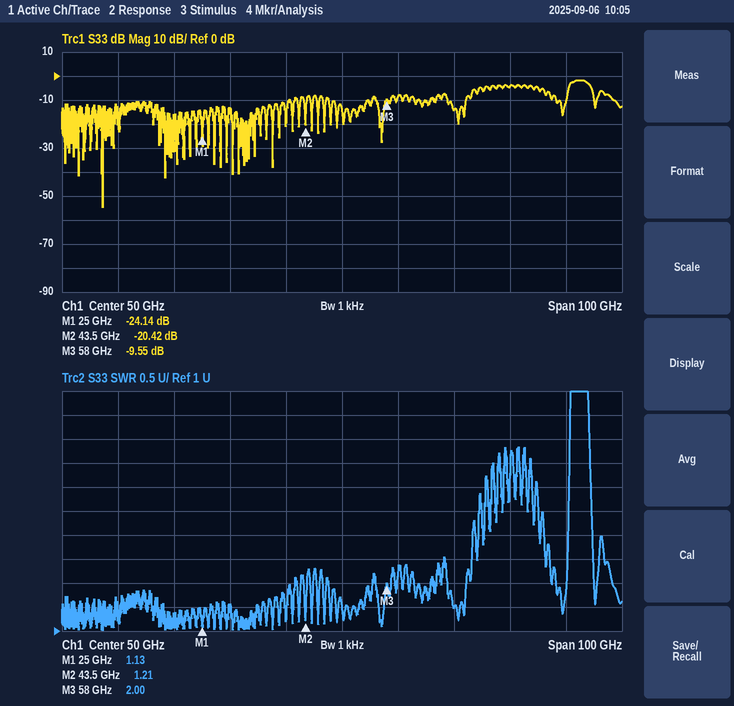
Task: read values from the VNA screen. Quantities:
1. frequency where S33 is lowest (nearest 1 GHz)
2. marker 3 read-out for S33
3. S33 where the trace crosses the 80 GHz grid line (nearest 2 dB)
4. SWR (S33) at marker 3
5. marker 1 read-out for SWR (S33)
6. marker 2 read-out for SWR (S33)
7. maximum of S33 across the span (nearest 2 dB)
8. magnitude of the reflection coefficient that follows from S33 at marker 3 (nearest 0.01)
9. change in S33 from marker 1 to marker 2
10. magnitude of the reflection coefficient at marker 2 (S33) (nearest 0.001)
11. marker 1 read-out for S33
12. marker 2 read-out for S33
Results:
7 GHz
-9.55 dB
-4 dB
2.00
1.13
1.21
-2 dB
0.33
3.72 dB
0.095
-24.14 dB
-20.42 dB
